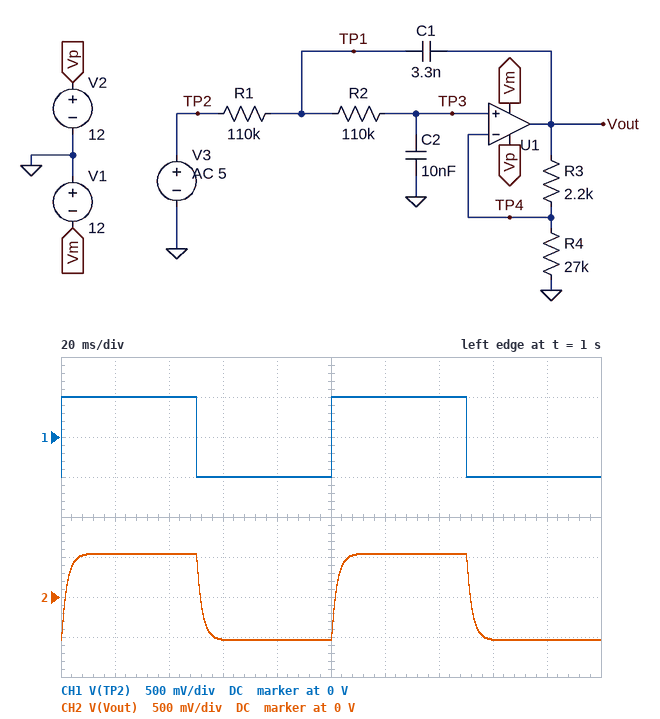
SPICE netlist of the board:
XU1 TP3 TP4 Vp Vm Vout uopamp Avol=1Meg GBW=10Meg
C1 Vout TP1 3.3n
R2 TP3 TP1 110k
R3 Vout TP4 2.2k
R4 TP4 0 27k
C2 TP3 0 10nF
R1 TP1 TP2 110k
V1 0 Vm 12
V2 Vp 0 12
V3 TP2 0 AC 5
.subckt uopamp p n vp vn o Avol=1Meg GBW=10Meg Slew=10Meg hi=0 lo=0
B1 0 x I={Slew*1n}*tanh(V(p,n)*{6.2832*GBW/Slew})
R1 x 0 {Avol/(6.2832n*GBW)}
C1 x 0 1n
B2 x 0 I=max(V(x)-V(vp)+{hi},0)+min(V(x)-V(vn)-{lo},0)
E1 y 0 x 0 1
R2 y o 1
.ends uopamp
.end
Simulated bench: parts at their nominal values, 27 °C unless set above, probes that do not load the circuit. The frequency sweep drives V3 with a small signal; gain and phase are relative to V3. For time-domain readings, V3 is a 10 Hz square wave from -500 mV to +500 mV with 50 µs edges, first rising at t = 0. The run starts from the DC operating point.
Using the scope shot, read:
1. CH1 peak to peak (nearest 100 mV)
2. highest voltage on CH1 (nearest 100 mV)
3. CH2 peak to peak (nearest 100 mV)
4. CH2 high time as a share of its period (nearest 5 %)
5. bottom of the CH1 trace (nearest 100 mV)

1.0 V
500 mV
1.1 V
50 %
-500 mV
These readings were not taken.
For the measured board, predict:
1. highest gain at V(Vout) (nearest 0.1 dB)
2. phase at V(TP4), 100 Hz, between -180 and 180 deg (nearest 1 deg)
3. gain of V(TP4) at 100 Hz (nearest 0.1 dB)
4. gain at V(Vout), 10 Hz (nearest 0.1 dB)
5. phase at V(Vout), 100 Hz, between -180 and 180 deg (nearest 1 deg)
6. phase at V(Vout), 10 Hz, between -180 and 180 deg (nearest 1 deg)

0.7 dB
-58 deg
-4.1 dB
0.6 dB
-58 deg
-8 deg
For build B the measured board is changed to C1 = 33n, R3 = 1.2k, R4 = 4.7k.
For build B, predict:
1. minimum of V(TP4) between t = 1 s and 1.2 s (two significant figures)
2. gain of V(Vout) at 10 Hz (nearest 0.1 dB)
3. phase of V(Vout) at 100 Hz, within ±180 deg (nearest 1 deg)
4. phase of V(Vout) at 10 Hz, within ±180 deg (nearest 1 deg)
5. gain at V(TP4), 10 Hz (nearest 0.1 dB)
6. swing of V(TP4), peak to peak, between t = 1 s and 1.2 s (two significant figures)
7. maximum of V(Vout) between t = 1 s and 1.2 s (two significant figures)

-850 mV
2.1 dB
-126 deg
-5 deg
0.1 dB
1.7 V
1.1 V
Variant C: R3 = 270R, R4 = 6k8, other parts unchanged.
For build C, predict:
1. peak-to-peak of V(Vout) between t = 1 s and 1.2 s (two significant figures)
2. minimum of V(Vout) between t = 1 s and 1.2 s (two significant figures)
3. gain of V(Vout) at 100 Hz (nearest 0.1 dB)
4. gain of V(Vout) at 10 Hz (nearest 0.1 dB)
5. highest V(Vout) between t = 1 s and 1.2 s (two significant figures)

1.0 V
-520 mV
-3.8 dB
0.3 dB
520 mV
